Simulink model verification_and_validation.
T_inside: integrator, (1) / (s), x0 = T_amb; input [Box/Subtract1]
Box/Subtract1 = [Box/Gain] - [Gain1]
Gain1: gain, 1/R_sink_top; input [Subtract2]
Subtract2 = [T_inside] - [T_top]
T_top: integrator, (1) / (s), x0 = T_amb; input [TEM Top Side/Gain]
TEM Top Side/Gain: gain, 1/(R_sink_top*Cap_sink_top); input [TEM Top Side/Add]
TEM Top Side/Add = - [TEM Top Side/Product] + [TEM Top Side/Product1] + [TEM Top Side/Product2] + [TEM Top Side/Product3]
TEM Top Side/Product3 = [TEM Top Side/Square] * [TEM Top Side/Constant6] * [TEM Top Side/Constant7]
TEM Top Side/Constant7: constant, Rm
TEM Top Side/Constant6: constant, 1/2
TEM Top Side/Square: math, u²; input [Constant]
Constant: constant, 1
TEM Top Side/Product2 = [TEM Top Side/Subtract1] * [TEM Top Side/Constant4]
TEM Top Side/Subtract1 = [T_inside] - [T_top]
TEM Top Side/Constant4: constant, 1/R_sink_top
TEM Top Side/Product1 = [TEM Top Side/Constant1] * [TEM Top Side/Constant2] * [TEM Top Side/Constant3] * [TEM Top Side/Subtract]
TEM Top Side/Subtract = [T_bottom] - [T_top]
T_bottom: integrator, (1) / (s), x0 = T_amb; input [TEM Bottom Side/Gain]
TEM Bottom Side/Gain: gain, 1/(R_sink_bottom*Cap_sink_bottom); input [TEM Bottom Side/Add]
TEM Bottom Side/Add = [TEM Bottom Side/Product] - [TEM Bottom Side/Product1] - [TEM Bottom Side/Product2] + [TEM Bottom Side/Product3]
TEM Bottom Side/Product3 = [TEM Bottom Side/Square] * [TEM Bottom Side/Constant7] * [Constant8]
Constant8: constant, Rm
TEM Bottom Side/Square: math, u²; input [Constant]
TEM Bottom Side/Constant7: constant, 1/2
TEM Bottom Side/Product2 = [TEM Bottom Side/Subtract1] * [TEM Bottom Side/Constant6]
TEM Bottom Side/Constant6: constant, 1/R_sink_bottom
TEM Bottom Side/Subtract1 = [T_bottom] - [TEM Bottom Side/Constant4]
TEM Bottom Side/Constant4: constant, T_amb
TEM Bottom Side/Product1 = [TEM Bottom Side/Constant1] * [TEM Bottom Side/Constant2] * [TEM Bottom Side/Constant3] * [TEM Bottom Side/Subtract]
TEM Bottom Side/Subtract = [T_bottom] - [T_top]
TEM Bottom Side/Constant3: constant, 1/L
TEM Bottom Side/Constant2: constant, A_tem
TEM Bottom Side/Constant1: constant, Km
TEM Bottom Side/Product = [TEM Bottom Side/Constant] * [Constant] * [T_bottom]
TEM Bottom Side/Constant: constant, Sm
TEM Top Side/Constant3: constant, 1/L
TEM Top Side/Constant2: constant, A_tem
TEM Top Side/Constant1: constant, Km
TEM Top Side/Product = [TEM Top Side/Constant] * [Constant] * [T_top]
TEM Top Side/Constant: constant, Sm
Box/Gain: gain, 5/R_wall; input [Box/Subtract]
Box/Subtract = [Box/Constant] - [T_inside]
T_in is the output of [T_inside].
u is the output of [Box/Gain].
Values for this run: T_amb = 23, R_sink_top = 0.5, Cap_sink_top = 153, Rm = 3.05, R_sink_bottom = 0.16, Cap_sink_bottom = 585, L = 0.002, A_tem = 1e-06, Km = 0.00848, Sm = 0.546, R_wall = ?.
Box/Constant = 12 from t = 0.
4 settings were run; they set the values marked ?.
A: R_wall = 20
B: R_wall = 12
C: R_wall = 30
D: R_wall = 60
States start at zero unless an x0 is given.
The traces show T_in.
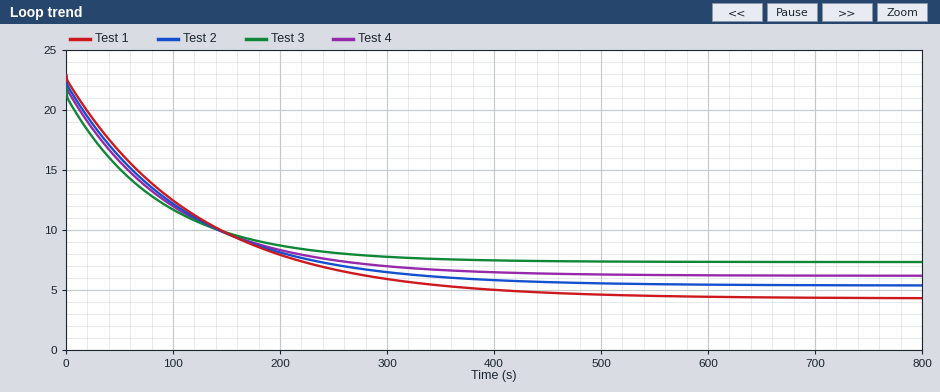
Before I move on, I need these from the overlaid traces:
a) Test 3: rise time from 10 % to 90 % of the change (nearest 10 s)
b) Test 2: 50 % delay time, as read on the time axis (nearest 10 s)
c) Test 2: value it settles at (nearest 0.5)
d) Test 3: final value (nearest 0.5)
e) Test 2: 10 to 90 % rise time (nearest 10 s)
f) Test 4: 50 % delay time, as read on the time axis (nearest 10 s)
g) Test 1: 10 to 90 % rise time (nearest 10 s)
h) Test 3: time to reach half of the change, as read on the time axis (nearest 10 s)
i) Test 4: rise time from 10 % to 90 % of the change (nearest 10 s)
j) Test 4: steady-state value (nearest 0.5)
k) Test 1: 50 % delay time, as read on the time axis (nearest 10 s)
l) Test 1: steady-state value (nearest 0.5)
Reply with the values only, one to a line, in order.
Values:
190 s
70 s
5.5
7.5
240 s
60 s
270 s
50 s
220 s
6.0
80 s
4.5
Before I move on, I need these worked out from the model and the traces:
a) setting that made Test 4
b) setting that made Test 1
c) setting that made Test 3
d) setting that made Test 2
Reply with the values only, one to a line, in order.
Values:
A
D
B
C
